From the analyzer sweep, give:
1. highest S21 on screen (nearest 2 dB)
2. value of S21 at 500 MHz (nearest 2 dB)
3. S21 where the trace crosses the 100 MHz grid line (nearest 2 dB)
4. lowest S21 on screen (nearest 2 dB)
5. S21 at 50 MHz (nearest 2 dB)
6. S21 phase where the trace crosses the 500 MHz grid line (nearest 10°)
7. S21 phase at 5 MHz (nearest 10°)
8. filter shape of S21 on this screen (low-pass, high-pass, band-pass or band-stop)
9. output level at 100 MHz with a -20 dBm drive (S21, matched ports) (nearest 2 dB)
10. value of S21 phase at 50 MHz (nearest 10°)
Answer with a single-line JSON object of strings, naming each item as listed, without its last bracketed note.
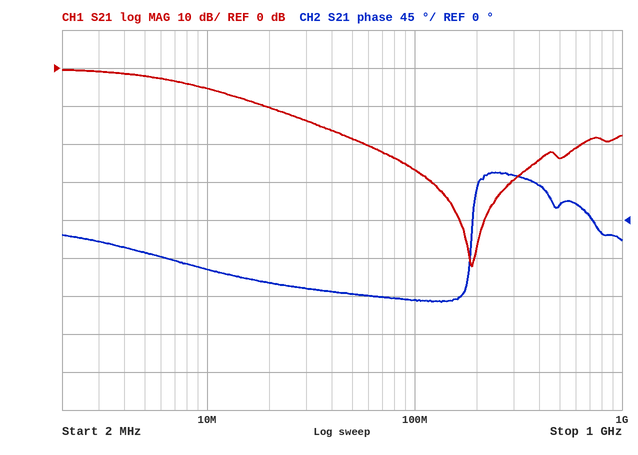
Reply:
{"highest S21 on screen": "0 dB", "value of S21 at 500 MHz": "-24 dB", "S21 where the trace crosses the 100 MHz grid line": "-26 dB", "lowest S21 on screen": "-52 dB", "S21 at 50 MHz": "-18 dB", "S21 phase where the trace crosses the 500 MHz grid line": "20°", "S21 phase at 5 MHz": "-40°", "filter shape of S21 on this screen": "low-pass", "output level at 100 MHz with a -20 dBm drive (S21, matched ports)": "-46 dBm", "value of S21 phase at 50 MHz": "-90°"}
